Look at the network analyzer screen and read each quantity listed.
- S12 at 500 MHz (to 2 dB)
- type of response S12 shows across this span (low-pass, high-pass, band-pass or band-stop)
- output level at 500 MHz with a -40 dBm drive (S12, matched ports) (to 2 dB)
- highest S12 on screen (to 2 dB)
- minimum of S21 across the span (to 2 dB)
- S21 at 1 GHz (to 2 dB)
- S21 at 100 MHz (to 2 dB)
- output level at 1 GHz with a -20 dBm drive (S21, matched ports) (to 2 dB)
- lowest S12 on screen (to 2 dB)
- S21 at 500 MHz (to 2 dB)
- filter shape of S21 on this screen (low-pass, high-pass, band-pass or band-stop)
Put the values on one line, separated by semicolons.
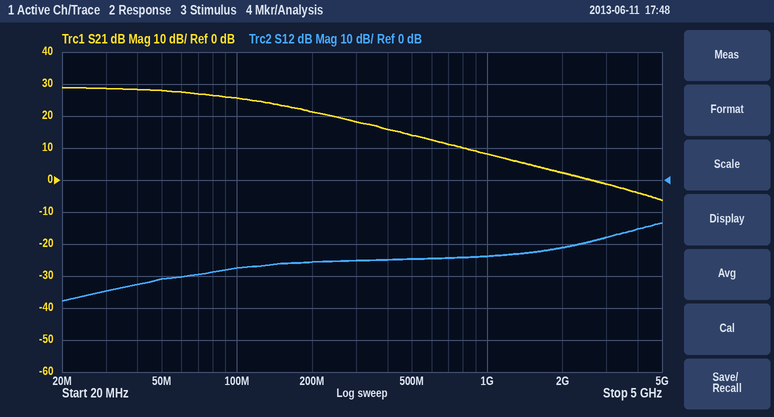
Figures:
-24 dB; high-pass; -64 dBm; -14 dB; -6 dB; 8 dB; 26 dB; -12 dBm; -38 dB; 14 dB; low-pass
